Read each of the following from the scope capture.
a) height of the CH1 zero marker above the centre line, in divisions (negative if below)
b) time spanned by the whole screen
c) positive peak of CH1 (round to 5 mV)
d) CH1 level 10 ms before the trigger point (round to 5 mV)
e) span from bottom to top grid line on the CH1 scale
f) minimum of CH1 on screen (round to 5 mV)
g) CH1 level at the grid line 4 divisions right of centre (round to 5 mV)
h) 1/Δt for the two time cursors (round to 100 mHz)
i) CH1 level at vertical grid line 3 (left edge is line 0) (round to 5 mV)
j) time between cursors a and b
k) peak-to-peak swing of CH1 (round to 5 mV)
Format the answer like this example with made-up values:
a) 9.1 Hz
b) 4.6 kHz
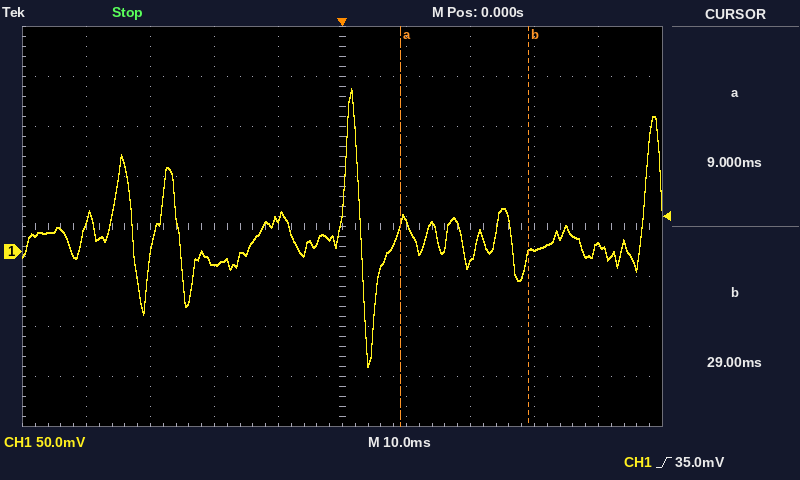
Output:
a) -0.5 div
b) 100 ms
c) 165 mV
d) 35 mV
e) 400 mV
f) -115 mV
g) 5 mV
h) 50.0 Hz
i) -15 mV
j) 20 ms
k) 280 mV
